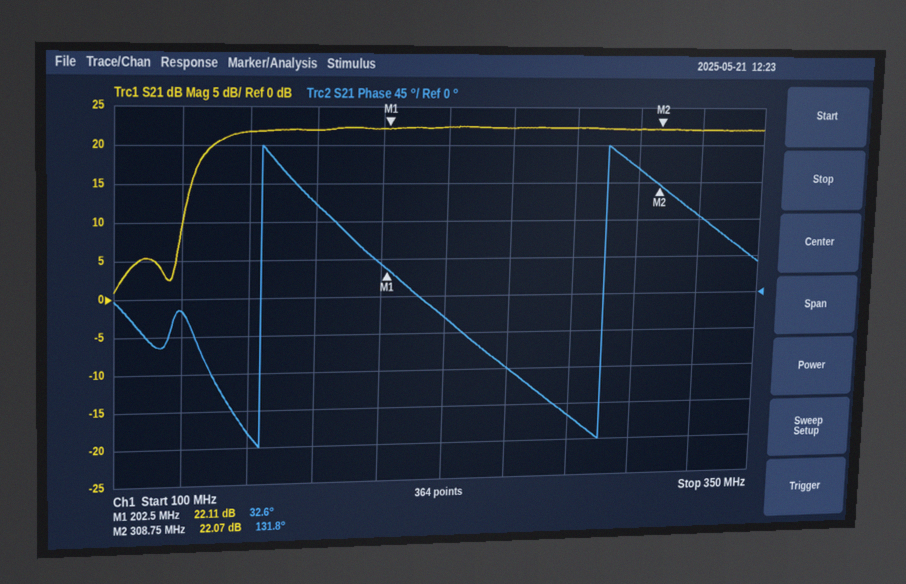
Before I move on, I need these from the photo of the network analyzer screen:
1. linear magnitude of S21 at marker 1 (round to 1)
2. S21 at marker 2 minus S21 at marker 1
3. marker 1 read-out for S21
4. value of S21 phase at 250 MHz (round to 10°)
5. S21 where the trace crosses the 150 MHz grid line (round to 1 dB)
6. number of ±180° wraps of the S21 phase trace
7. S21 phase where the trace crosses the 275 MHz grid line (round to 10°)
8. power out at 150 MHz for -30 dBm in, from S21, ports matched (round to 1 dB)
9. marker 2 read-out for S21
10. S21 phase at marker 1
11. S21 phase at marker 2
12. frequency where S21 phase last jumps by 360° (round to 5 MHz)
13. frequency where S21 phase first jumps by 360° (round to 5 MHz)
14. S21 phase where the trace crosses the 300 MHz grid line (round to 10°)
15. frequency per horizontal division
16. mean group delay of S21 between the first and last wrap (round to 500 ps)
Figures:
13
-0.04 dB
22.11 dB
-90°
22 dB
2
-150°
-8 dBm
22.07 dB
32.6°
131.8°
290 MHz
155 MHz
150°
25 MHz
7.5 ns
